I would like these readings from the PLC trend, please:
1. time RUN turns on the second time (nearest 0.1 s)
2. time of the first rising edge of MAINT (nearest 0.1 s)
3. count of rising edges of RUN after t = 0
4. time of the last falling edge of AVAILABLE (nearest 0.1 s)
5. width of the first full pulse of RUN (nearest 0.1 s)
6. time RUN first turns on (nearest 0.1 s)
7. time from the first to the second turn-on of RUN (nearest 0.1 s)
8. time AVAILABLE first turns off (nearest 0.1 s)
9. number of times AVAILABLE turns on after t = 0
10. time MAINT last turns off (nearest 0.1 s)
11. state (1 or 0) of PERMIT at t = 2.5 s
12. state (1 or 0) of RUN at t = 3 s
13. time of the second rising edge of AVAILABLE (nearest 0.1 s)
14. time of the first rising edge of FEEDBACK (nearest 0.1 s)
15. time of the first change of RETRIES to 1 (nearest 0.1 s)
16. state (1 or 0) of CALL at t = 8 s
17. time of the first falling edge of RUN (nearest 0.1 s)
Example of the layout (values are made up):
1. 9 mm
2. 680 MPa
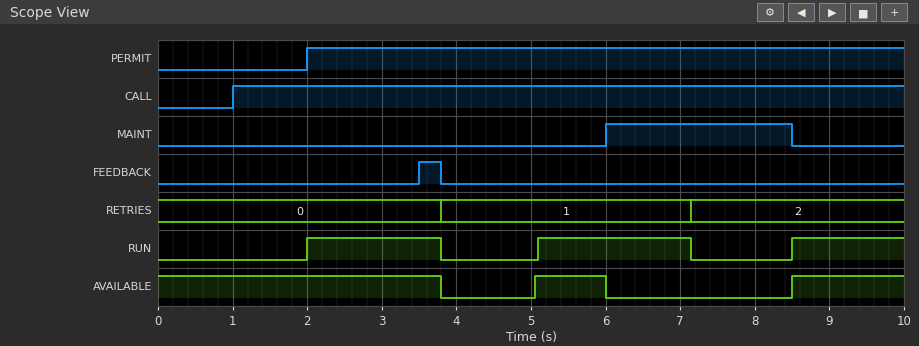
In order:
1. 5.1 s
2. 6.0 s
3. 3
4. 6.0 s
5. 1.8 s
6. 2.0 s
7. 3.1 s
8. 3.8 s
9. 2
10. 8.5 s
11. 1
12. 1
13. 8.5 s
14. 3.5 s
15. 3.8 s
16. 1
17. 3.8 s
